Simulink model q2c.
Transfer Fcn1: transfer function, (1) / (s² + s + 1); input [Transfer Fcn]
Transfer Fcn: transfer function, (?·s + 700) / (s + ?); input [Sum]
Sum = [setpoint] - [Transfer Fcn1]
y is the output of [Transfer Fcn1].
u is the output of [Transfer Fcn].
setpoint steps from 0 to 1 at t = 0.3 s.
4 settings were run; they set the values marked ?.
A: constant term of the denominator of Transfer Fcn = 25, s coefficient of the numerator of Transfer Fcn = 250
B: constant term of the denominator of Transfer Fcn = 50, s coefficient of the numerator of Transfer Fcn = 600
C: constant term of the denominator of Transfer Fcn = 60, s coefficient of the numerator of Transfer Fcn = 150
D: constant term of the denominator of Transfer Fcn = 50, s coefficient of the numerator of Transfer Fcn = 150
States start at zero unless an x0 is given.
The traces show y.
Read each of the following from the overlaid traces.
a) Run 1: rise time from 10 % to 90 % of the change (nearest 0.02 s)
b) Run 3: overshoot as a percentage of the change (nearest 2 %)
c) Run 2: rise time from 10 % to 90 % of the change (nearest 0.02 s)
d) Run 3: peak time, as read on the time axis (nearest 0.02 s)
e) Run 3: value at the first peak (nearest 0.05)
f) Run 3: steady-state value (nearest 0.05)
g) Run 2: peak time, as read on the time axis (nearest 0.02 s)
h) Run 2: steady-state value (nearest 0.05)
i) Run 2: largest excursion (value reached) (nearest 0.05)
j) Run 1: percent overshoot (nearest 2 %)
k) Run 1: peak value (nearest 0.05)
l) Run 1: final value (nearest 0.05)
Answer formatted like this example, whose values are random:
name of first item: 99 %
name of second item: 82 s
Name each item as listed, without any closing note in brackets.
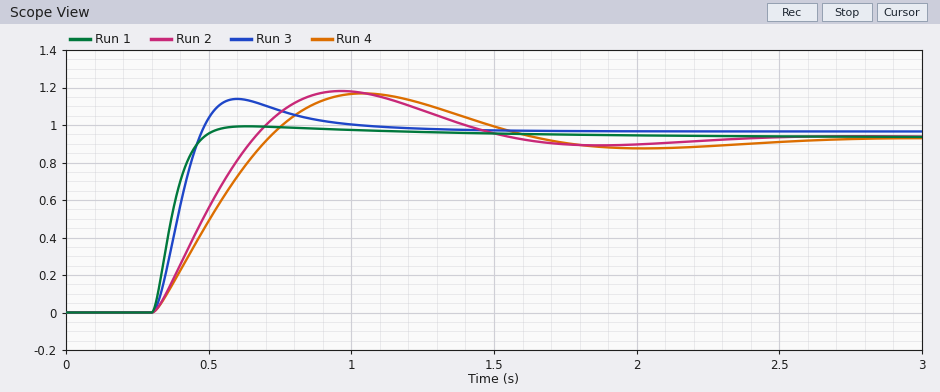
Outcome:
Run 1: rise time from 10 % to 90 % of the change: 0.12 s
Run 3: overshoot as a percentage of the change: 18 %
Run 2: rise time from 10 % to 90 % of the change: 0.26 s
Run 3: peak time, as read on the time axis: 0.60 s
Run 3: value at the first peak: 1.15
Run 3: steady-state value: 0.95
Run 2: peak time, as read on the time axis: 0.96 s
Run 2: steady-state value: 0.95
Run 2: largest excursion (value reached): 1.20
Run 1: percent overshoot: 6 %
Run 1: peak value: 1.00
Run 1: final value: 0.95
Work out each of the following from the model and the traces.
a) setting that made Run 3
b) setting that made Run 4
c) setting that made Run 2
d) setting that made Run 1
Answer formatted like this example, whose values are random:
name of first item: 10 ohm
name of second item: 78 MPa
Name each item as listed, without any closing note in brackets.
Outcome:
setting that made Run 3: A
setting that made Run 4: C
setting that made Run 2: D
setting that made Run 1: B
